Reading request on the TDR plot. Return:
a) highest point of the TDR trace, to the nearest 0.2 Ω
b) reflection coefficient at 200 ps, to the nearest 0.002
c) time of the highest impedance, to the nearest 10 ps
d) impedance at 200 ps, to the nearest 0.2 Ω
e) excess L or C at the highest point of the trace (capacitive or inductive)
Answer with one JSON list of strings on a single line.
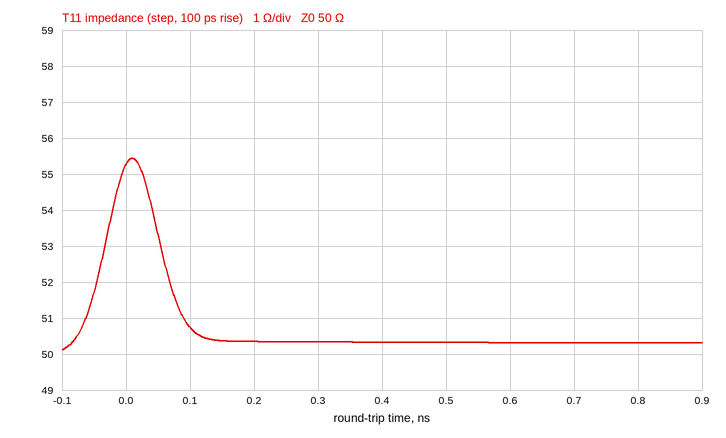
["55.4 Ω", "+0.004", "10 ps", "50.4 Ω", "inductive"]
